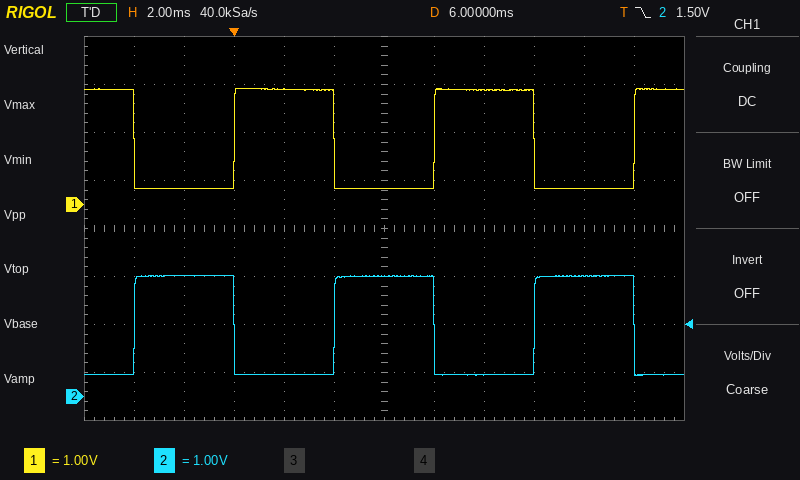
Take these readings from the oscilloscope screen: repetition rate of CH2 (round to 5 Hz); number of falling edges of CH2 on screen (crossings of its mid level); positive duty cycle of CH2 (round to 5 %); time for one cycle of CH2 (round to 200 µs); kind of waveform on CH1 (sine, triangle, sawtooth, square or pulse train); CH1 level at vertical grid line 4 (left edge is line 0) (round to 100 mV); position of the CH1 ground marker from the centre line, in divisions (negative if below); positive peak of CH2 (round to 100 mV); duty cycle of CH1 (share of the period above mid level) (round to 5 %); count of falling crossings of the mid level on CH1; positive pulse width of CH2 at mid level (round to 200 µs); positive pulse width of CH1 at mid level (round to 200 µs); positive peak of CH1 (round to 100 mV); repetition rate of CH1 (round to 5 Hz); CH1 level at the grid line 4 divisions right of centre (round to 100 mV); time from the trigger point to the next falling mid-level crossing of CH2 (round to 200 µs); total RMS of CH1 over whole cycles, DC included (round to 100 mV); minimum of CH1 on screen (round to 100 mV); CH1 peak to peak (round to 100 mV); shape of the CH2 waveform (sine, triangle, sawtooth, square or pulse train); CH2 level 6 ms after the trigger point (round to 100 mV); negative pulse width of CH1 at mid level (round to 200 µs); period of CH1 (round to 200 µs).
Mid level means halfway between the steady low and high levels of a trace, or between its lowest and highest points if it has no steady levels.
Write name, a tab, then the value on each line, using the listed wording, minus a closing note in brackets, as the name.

repetition rate of CH2	125 Hz
number of falling edges of CH2 on screen	3
positive duty cycle of CH2	50 %
time for one cycle of CH2	8.0 ms
kind of waveform on CH1	square
CH1 level at vertical grid line 4 (left edge is line 0)	2.4 V
position of the CH1 ground marker from the centre line, in divisions	+0.5 div
positive peak of CH2	2.5 V
duty cycle of CH1 (share of the period above mid level)	50 %
count of falling crossings of the mid level on CH1	3
positive pulse width of CH2 at mid level	4.0 ms
positive pulse width of CH1 at mid level	4.0 ms
positive peak of CH1	2.4 V
repetition rate of CH1	125 Hz
CH1 level at the grid line 4 divisions right of centre	300 mV
time from the trigger point to the next falling mid-level crossing of CH2	8.0 ms
total RMS of CH1 over whole cycles, DC included	1.7 V
minimum of CH1 on screen	300 mV
CH1 peak to peak	2.1 V
shape of the CH2 waveform	square
CH2 level 6 ms after the trigger point	2.5 V
negative pulse width of CH1 at mid level	4.0 ms
period of CH1	8.0 ms
